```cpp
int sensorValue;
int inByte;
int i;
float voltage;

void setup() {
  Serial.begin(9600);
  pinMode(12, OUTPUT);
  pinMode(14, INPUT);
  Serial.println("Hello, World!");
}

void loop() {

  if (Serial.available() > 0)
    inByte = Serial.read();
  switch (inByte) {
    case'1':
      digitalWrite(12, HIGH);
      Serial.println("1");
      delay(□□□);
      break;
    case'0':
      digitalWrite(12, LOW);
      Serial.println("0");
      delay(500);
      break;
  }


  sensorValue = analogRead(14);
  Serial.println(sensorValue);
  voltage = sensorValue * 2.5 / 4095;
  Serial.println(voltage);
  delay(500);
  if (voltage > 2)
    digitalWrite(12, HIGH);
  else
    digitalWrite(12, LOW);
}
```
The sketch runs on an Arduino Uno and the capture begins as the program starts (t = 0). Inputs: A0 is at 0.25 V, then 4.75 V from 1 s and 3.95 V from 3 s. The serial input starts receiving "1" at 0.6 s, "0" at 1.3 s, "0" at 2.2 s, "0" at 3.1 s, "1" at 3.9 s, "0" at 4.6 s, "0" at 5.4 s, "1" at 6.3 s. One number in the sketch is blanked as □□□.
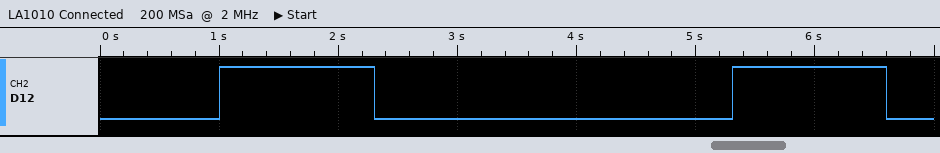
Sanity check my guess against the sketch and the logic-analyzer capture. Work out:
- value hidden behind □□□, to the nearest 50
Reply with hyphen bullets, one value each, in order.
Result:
- 800
